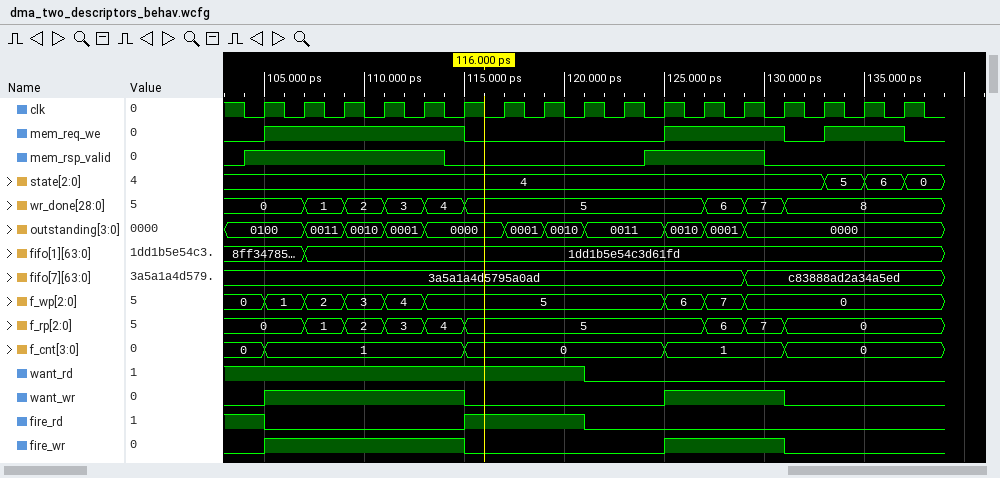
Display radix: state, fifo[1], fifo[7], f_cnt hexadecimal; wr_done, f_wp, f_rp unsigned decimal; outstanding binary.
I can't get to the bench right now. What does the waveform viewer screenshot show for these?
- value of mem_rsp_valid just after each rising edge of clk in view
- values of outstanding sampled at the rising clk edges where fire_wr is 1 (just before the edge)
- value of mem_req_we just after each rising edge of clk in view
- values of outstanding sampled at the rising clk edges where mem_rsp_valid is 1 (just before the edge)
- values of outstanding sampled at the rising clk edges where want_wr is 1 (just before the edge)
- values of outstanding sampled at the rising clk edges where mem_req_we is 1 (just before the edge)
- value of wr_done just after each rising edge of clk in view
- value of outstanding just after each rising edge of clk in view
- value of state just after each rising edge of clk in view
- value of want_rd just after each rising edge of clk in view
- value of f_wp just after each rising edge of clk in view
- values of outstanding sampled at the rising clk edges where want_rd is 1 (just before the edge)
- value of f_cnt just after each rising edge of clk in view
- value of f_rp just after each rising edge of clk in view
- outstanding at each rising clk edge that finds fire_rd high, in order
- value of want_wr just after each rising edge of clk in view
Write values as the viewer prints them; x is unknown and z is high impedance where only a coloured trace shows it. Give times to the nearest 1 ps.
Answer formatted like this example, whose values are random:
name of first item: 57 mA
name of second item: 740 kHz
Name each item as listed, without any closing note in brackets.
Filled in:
value of mem_rsp_valid just after each rising edge of clk in view: 1 1 1 1 1 0 0 0 0 0 1 1 1 0 0 0 0
values of outstanding sampled at the rising clk edges where fire_wr is 1: 0100, 0011, 0010, 0001, 0000, 0010, 0001, 0000
value of mem_req_we just after each rising edge of clk in view: 1 1 1 1 1 0 0 0 0 0 1 1 1 0 1 1 0
values of outstanding sampled at the rising clk edges where mem_rsp_valid is 1: 0100, 0100, 0011, 0010, 0001, 0011, 0010, 0001
values of outstanding sampled at the rising clk edges where want_wr is 1: 0100, 0011, 0010, 0001, 0000, 0010, 0001, 0000
values of outstanding sampled at the rising clk edges where mem_req_we is 1: 0100, 0011, 0010, 0001, 0000, 0010, 0001, 0000, 0000, 0000
value of wr_done just after each rising edge of clk in view: 0, 1, 2, 3, 4, 5, 5, 5, 5, 5, 5, 6, 7, 8, 8, 8, 8
value of outstanding just after each rising edge of clk in view: 0100, 0011, 0010, 0001, 0000, 0000, 0001, 0010, 0011, 0011, 0010, 0001, 0000, 0000, 0000, 0000, 0000
value of state just after each rising edge of clk in view: 4, 4, 4, 4, 4, 4, 4, 4, 4, 4, 4, 4, 4, 4, 5, 6, 0
value of want_rd just after each rising edge of clk in view: 1 1 1 1 1 1 1 1 0 0 0 0 0 0 0 0 0
value of f_wp just after each rising edge of clk in view: 1, 2, 3, 4, 5, 5, 5, 5, 5, 5, 6, 7, 0, 0, 0, 0, 0
values of outstanding sampled at the rising clk edges where want_rd is 1: 0100, 0100, 0011, 0010, 0001, 0000, 0000, 0001, 0010
value of f_cnt just after each rising edge of clk in view: 1, 1, 1, 1, 1, 0, 0, 0, 0, 0, 1, 1, 1, 0, 0, 0, 0
value of f_rp just after each rising edge of clk in view: 0, 1, 2, 3, 4, 5, 5, 5, 5, 5, 5, 6, 7, 0, 0, 0, 0
outstanding at each rising clk edge that finds fire_rd high, in order: 0100, 0000, 0001, 0010
value of want_wr just after each rising edge of clk in view: 1 1 1 1 1 0 0 0 0 0 1 1 1 0 0 0 0
